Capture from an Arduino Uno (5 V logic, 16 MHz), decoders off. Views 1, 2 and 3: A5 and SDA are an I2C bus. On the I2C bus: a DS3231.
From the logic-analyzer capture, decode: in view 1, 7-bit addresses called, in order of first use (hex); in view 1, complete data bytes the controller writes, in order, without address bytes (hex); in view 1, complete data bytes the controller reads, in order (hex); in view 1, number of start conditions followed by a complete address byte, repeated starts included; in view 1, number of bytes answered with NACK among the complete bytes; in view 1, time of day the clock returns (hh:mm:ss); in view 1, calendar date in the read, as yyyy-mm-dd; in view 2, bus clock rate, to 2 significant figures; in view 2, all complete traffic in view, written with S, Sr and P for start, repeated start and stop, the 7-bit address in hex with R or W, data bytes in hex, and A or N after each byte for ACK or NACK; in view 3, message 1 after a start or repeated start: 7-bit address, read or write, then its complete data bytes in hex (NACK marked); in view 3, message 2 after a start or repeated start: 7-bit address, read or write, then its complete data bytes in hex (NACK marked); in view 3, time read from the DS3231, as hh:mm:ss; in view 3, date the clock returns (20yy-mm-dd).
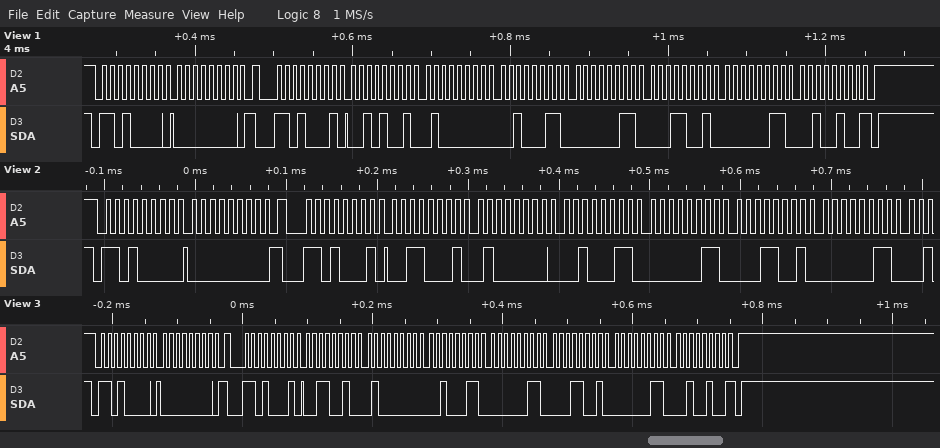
0x68
00
29 40 23 03 19 03 24
2
1
23:40:29
2024-03-19
100 kHz
S 68W A 00 A Sr 68R A 31 A 40 A 23 A 03 A 19 A 03 A
0x68 write: 00
0x68 read: 32 40 23 03 19 03 24 NACK
23:40:32
2024-03-19
